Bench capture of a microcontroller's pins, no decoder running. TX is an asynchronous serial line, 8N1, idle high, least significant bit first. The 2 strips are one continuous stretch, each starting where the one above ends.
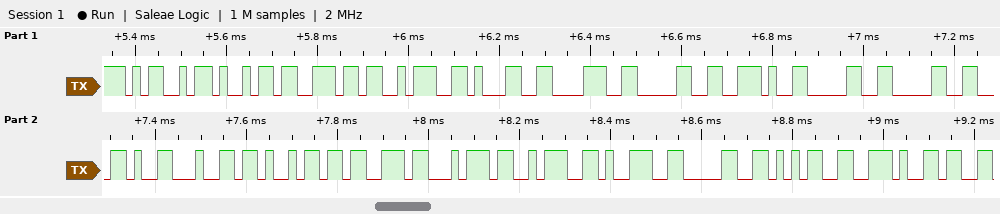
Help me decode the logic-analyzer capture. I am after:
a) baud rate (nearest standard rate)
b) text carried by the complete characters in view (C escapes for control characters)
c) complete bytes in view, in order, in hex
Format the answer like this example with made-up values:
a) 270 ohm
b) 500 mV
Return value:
a) 57600 baud
b) "Min:180.00,dist:905."
c) 4D 69 6E 3A 31 38 30 2E 30 30 2C 64 69 73 74 3A 39 30 35 2E
